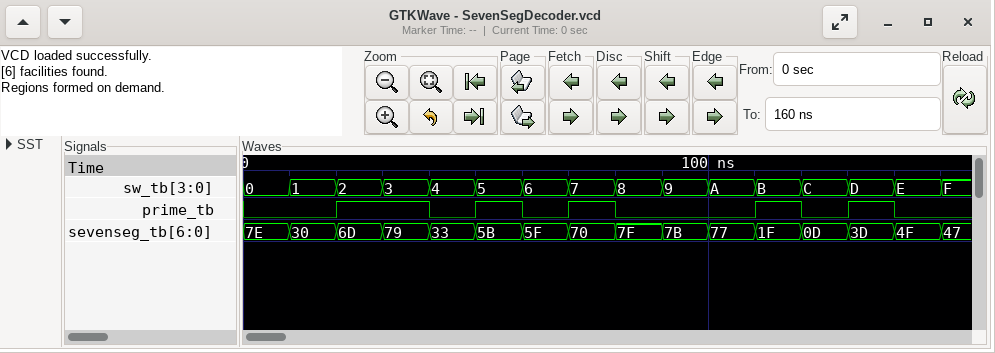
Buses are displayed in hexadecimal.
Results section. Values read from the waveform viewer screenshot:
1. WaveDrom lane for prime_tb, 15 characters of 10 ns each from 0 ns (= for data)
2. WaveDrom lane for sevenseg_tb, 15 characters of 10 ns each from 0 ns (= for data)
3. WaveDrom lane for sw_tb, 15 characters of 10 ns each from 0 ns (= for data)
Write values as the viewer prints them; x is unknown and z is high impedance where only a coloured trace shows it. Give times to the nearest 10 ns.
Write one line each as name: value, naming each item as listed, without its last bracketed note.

WaveDrom lane for prime_tb, 15 characters of 10 ns each from 0 ns: {name: 'prime_tb', wave: '0.1.01010..1010'}
WaveDrom lane for sevenseg_tb, 15 characters of 10 ns each from 0 ns: {name: 'sevenseg_tb', wave: '===============', data: '7E 30 6D 79 33 5B 5F 70 7F 7B 77 1F 0D 3D 4F'}
WaveDrom lane for sw_tb, 15 characters of 10 ns each from 0 ns: {name: 'sw_tb', wave: '===============', data: '0 1 2 3 4 5 6 7 8 9 A B C D E'}
